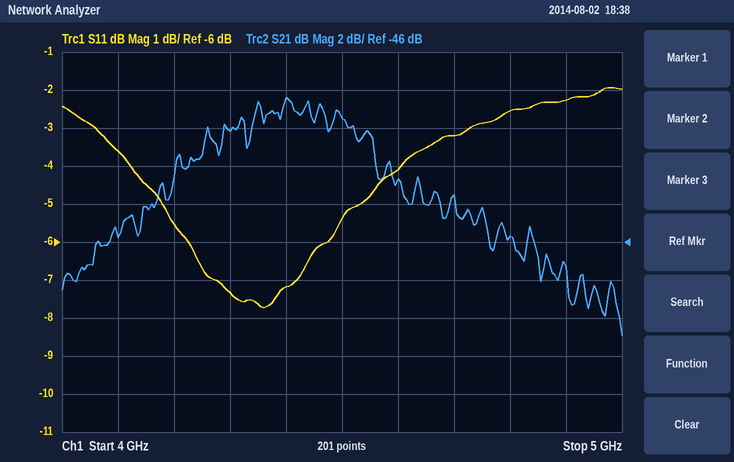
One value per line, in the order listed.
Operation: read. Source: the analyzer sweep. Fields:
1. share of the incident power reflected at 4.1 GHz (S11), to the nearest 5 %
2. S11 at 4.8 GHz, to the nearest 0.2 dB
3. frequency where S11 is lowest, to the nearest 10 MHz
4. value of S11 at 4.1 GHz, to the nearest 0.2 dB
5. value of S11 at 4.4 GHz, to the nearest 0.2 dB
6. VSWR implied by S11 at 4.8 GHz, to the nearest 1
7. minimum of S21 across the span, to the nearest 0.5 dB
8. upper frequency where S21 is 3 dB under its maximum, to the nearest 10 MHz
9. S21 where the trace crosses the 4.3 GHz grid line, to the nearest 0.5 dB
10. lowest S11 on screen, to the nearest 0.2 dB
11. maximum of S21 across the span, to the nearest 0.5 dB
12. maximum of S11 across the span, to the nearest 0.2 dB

45 %
-2.6 dB
4.36 GHz
-3.6 dB
-7.2 dB
7
-51.0 dB
4.56 GHz
-40.0 dB
-7.8 dB
-38.5 dB
-2.0 dB
